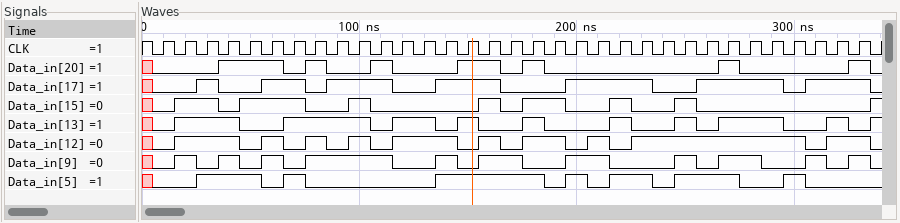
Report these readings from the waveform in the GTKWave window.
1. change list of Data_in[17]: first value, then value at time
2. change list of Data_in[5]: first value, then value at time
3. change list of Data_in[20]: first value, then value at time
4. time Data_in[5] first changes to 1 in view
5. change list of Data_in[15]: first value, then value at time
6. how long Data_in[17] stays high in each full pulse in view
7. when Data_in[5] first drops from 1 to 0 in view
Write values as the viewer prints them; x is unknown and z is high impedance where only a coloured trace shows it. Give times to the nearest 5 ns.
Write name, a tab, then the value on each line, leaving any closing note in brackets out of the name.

change list of Data_in[17]: first value, then value at time	x, 0 at 5 ns, 1 at 25 ns, 0 at 35 ns, 1 at 55 ns, 0 at 75 ns, 1 at 85 ns, 0 at 115 ns, 1 at 135 ns, 0 at 165 ns, 1 at 195 ns, 0 at 235 ns, 1 at 255 ns, 0 at 295 ns, 1 at 305 ns, 0 at 335 ns
change list of Data_in[5]: first value, then value at time	x, 0 at 5 ns, 1 at 25 ns, 0 at 55 ns, 1 at 65 ns, 0 at 75 ns, 1 at 135 ns, 0 at 185 ns, 1 at 195 ns, 0 at 205 ns, 1 at 215 ns, 0 at 235 ns, 1 at 245 ns, 0 at 275 ns, 1 at 295 ns, 0 at 305 ns
change list of Data_in[20]: first value, then value at time	x, 0 at 5 ns, 1 at 35 ns, 0 at 65 ns, 1 at 75 ns, 0 at 85 ns, 1 at 105 ns, 0 at 115 ns, 1 at 145 ns, 0 at 165 ns, 1 at 175 ns, 0 at 185 ns, 1 at 265 ns, 0 at 275 ns, 1 at 325 ns, 0 at 335 ns
time Data_in[5] first changes to 1 in view	25 ns
change list of Data_in[15]: first value, then value at time	x, 0 at 5 ns, 1 at 15 ns, 0 at 35 ns, 1 at 45 ns, 0 at 75 ns, 1 at 95 ns, 0 at 105 ns, 1 at 155 ns, 0 at 165 ns, 1 at 175 ns, 0 at 195 ns, 1 at 215 ns, 0 at 225 ns, 1 at 245 ns, 0 at 255 ns, 1 at 335 ns
how long Data_in[17] stays high in each full pulse in view	10 ns, 20 ns, 30 ns, 30 ns, 40 ns, 40 ns, 30 ns
when Data_in[5] first drops from 1 to 0 in view	55 ns
